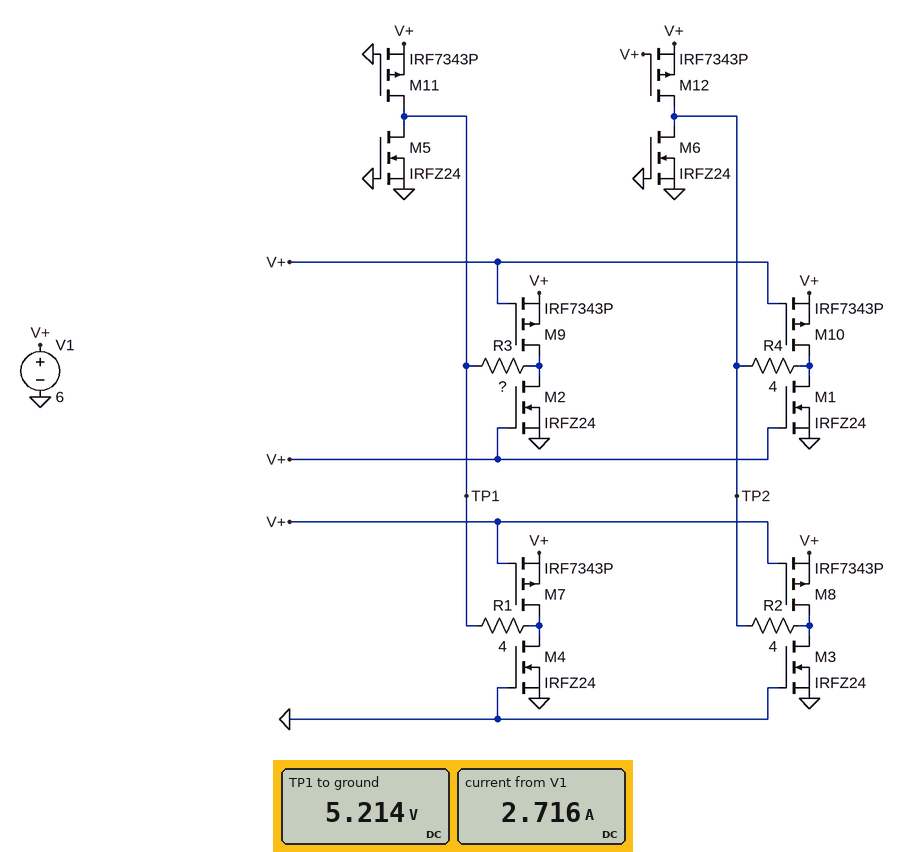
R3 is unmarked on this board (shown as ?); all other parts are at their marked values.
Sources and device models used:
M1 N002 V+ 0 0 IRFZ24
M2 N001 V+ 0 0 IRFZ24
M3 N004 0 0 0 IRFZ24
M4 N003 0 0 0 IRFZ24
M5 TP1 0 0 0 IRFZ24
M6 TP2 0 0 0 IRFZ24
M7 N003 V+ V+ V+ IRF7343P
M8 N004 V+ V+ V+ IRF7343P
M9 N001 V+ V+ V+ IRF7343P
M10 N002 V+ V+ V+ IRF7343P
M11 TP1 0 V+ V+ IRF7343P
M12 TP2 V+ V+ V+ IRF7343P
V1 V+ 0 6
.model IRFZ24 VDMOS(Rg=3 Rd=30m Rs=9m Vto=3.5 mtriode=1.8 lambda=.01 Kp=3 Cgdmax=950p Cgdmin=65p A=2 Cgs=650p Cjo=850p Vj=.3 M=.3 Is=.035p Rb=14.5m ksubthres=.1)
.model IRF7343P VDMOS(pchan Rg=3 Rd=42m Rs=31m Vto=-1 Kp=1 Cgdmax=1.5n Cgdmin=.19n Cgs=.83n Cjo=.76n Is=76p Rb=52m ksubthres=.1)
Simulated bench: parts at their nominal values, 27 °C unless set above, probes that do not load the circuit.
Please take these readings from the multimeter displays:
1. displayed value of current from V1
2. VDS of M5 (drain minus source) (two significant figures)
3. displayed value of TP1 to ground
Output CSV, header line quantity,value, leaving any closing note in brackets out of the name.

quantity,value
displayed value of current from V1,2.716 A
VDS of M5 (drain minus source),5.2 V
displayed value of TP1 to ground,5.214 V
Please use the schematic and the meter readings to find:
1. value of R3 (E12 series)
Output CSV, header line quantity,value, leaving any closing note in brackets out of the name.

quantity,value
value of R3,1.8 Ω
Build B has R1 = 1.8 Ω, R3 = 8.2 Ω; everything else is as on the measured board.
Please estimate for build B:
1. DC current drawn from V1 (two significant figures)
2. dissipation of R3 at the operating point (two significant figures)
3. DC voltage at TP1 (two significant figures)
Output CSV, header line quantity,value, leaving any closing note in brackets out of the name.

quantity,value
DC current drawn from V1,700 mA
dissipation of R3 at the operating point,4.0 W
DC voltage at TP1,5.8 V
